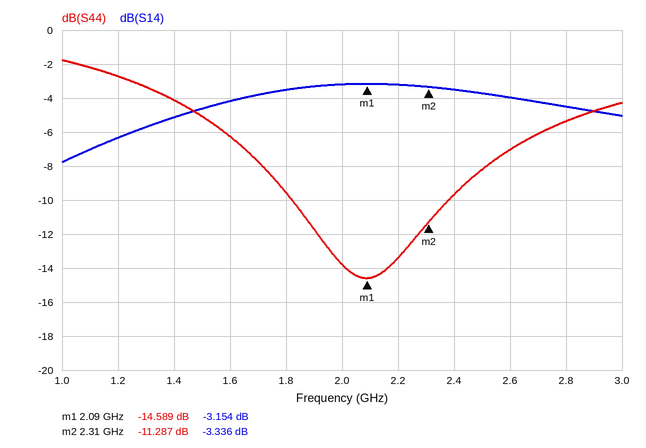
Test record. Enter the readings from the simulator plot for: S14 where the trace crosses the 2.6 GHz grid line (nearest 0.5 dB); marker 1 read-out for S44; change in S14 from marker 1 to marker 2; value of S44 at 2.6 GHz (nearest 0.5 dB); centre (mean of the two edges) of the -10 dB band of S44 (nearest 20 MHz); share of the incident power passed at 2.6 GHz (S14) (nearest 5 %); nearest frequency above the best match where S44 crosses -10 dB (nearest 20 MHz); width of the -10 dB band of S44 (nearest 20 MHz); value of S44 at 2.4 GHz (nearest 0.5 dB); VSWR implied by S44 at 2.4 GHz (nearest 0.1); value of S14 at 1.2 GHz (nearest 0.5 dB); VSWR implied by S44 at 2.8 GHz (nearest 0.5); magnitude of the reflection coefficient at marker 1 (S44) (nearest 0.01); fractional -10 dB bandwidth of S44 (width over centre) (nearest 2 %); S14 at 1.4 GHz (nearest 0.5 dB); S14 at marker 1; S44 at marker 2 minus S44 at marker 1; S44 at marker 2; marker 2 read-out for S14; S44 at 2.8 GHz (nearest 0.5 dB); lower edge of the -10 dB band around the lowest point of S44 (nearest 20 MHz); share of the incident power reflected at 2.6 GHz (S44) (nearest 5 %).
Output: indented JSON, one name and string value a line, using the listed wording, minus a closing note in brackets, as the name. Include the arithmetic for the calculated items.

{
  "S14 where the trace crosses the 2.6 GHz grid line": "-4.0 dB",
  "marker 1 read-out for S44": "-14.589 dB",
  "change in S14 from marker 1 to marker 2": "-3.336 − (-3.154) = -0.182 dB",
  "value of S44 at 2.6 GHz": "-7.0 dB",
  "centre (mean of the two edges) of the -10 dB band of S44": "2.10 GHz",
  "share of the incident power passed at 2.6 GHz (S14)": "10^(-4/10) ≈ 40 %",
  "nearest frequency above the best match where S44 crosses -10 dB": "2.38 GHz",
  "width of the -10 dB band of S44": "2.38 GHz − 1.82 GHz = 560 MHz",
  "value of S44 at 2.4 GHz": "-9.5 dB",
  "VSWR implied by S44 at 2.4 GHz": "|Γ| = 10^(-9.5/20) = 0.3350; VSWR = (1 + 0.3350)/(1 − 0.3350) ≈ 2.0",
  "value of S14 at 1.2 GHz": "-6.5 dB",
  "VSWR implied by S44 at 2.8 GHz": "|Γ| = 10^(-5.5/20) = 0.5309; VSWR = (1 + 0.5309)/(1 − 0.5309) ≈ 3.26, so 3.5 to the nearest 0.5",
  "magnitude of the reflection coefficient at marker 1 (S44)": "10^(-14.589/20) ≈ 0.19",
  "fractional -10 dB bandwidth of S44 (width over centre)": "560 MHz / 2.1 GHz ≈ 26.7 %, so 26 % to the nearest 2 %",
  "S14 at 1.4 GHz": "-5.0 dB",
  "S14 at marker 1": "-3.154 dB",
  "S44 at marker 2 minus S44 at marker 1": "-11.287 − (-14.589) = 3.302 dB",
  "S44 at marker 2": "-11.287 dB",
  "marker 2 read-out for S14": "-3.336 dB",
  "S44 at 2.8 GHz": "-5.5 dB",
  "lower edge of the -10 dB band around the lowest point of S44": "1.82 GHz",
  "share of the incident power reflected at 2.6 GHz (S44)": "10^(-7/10) ≈ 20 %"
}
